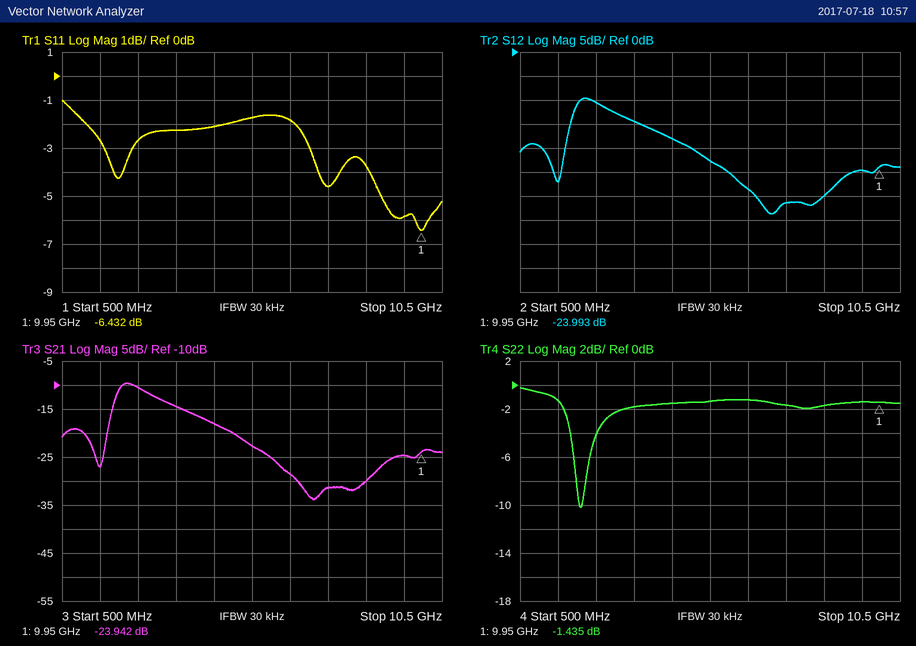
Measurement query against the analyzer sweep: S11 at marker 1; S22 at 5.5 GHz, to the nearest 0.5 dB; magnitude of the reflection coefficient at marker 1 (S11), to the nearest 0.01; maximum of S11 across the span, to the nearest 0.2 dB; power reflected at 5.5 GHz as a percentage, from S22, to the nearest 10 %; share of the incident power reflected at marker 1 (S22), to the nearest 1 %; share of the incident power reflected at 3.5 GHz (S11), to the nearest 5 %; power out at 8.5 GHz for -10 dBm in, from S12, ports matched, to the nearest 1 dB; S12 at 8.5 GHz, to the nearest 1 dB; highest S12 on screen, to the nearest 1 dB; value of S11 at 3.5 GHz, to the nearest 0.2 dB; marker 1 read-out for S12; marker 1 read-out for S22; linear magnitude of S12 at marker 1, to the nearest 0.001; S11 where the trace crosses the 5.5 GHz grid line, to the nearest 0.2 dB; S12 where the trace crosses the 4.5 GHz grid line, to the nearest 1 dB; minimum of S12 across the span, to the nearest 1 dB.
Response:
-6.432 dB
-1.5 dB
0.48
-1.0 dB
70 %
72 %
60 %
-40 dBm
-30 dB
-10 dB
-2.2 dB
-23.993 dB
-1.435 dB
0.063
-1.8 dB
-18 dB
-34 dB
